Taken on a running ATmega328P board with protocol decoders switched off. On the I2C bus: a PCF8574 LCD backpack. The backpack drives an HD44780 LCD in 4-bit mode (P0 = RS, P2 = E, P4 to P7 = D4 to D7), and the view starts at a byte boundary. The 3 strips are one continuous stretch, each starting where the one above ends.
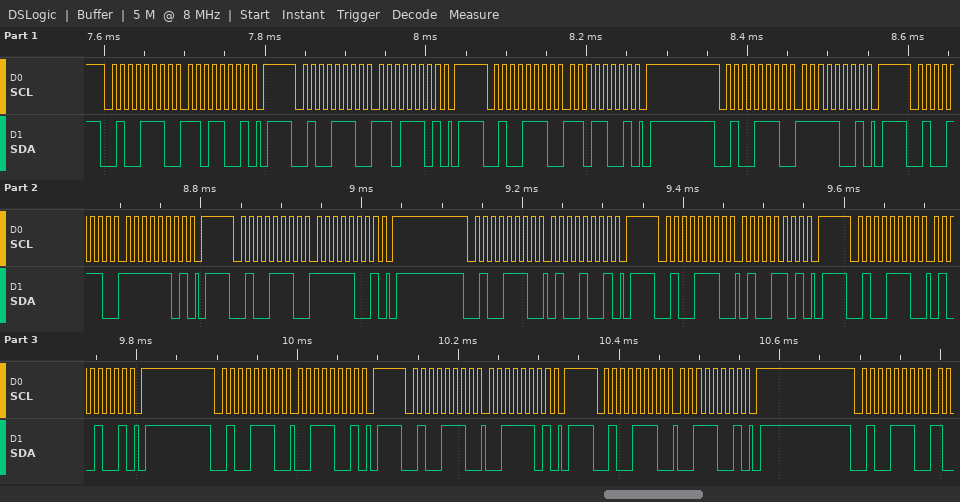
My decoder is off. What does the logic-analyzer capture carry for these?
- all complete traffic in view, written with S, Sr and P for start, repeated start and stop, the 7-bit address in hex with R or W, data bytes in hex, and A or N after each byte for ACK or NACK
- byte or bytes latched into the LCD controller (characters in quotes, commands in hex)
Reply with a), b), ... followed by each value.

a) S 27W A D9 A P S 27W A DD A P S 27W A D9 A P S 27W A F9 A P S 27W A FD A P S 27W A F9 A P S 27W A 49 A P S 27W A 4D A P S 27W A 49 A P S 27W A 39 A P S 27W A 3D A P S 27W A 39 A P S 27W A
b) data 0xDF 'C'
